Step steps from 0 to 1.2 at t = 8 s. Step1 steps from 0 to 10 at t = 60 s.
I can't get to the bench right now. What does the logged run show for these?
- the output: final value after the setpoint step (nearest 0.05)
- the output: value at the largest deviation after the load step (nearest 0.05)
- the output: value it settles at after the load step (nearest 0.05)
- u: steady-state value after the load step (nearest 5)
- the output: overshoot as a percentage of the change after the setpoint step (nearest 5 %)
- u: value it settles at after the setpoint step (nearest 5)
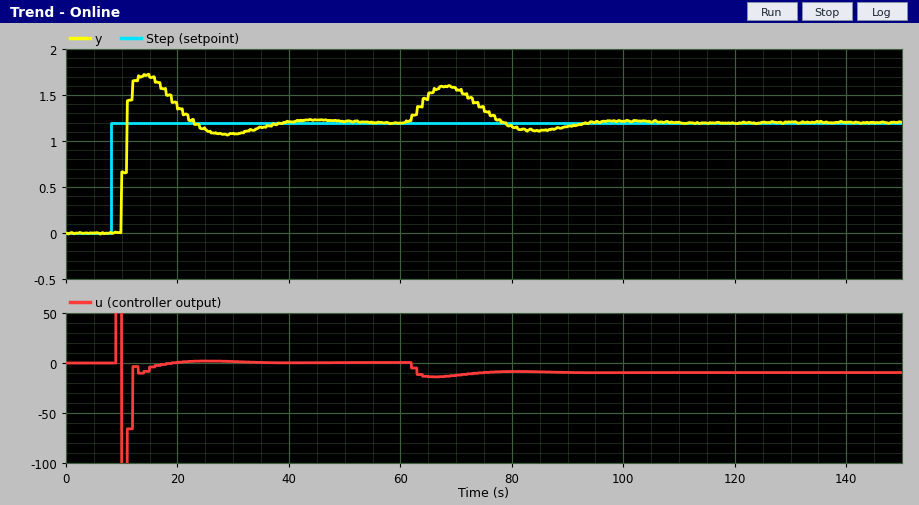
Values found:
1.20
1.60
1.20
-10
45 %
0
